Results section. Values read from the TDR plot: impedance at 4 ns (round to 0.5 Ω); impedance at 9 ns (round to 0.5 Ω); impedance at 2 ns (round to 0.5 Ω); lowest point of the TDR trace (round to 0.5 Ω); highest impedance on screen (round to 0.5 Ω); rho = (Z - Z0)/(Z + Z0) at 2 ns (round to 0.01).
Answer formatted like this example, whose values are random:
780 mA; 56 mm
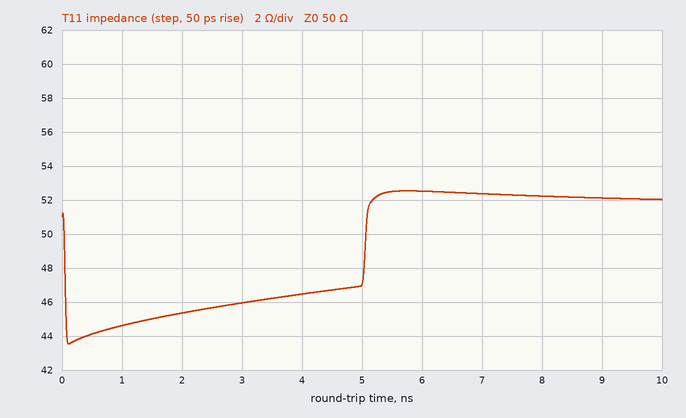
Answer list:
46.5 Ω; 52.0 Ω; 45.5 Ω; 43.5 Ω; 52.5 Ω; -0.05
